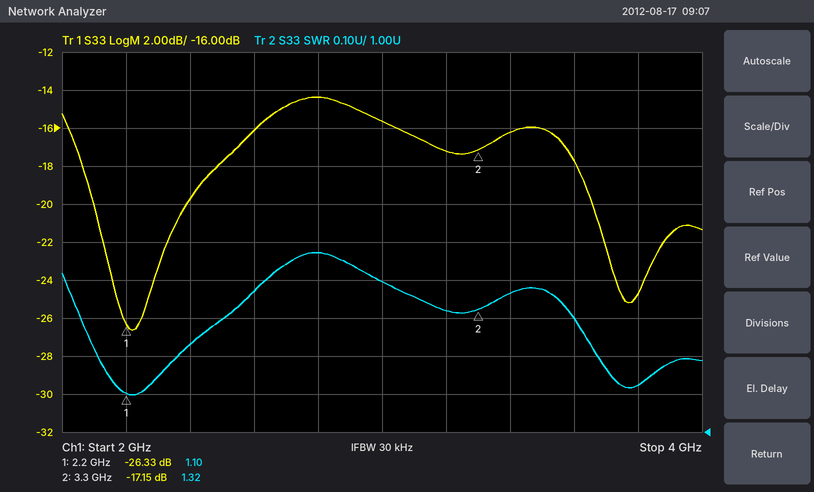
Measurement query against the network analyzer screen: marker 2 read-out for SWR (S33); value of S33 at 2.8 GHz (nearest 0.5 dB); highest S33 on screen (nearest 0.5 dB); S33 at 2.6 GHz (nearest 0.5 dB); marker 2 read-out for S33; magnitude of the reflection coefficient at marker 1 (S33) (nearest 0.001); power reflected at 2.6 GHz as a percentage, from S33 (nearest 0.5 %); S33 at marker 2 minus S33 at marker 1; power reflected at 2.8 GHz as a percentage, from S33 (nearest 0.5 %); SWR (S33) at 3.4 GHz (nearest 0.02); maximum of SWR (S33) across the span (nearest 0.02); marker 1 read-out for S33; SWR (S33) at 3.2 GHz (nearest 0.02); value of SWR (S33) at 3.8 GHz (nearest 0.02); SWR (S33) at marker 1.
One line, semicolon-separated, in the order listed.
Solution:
1.32; -14.5 dB; -14.5 dB; -16.0 dB; -17.15 dB; 0.048; 2.5 %; 9.18 dB; 3.5 %; 1.36; 1.48; -26.33 dB; 1.32; 1.12; 1.10
